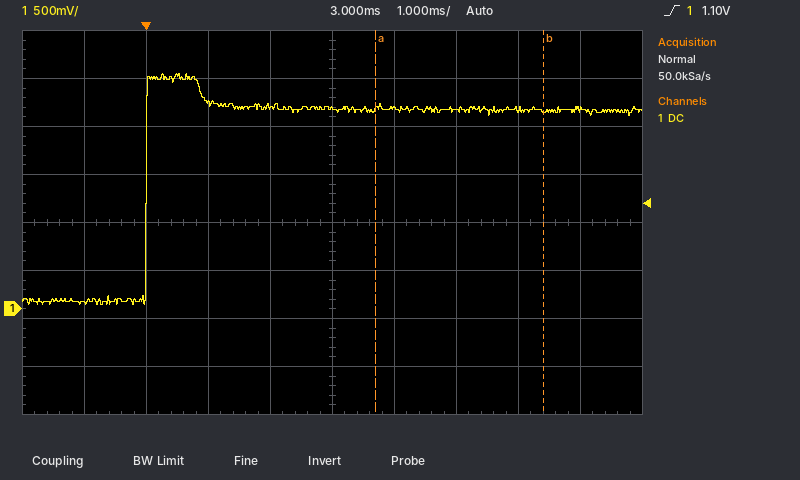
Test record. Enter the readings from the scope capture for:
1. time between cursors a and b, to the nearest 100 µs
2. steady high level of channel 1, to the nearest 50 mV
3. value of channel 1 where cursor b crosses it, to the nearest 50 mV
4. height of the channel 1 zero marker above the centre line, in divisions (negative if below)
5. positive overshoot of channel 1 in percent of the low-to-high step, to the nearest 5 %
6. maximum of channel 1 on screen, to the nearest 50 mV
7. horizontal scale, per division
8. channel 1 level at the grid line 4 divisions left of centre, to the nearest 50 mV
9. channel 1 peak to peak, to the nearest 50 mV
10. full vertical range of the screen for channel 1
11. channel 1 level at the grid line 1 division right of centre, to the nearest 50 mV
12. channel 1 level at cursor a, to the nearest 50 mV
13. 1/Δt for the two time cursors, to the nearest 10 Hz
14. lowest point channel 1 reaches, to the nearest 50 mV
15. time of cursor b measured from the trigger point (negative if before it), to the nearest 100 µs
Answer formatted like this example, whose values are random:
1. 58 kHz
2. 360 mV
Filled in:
1. 2.7 ms
2. 2.10 V
3. 2.05 V
4. -1.8 div
5. 20 %
6. 2.45 V
7. 1 ms
8. 50 mV
9. 2.40 V
10. 4 V
11. 2.10 V
12. 2.10 V
13. 370 Hz
14. 50 mV
15. +6.4 ms
